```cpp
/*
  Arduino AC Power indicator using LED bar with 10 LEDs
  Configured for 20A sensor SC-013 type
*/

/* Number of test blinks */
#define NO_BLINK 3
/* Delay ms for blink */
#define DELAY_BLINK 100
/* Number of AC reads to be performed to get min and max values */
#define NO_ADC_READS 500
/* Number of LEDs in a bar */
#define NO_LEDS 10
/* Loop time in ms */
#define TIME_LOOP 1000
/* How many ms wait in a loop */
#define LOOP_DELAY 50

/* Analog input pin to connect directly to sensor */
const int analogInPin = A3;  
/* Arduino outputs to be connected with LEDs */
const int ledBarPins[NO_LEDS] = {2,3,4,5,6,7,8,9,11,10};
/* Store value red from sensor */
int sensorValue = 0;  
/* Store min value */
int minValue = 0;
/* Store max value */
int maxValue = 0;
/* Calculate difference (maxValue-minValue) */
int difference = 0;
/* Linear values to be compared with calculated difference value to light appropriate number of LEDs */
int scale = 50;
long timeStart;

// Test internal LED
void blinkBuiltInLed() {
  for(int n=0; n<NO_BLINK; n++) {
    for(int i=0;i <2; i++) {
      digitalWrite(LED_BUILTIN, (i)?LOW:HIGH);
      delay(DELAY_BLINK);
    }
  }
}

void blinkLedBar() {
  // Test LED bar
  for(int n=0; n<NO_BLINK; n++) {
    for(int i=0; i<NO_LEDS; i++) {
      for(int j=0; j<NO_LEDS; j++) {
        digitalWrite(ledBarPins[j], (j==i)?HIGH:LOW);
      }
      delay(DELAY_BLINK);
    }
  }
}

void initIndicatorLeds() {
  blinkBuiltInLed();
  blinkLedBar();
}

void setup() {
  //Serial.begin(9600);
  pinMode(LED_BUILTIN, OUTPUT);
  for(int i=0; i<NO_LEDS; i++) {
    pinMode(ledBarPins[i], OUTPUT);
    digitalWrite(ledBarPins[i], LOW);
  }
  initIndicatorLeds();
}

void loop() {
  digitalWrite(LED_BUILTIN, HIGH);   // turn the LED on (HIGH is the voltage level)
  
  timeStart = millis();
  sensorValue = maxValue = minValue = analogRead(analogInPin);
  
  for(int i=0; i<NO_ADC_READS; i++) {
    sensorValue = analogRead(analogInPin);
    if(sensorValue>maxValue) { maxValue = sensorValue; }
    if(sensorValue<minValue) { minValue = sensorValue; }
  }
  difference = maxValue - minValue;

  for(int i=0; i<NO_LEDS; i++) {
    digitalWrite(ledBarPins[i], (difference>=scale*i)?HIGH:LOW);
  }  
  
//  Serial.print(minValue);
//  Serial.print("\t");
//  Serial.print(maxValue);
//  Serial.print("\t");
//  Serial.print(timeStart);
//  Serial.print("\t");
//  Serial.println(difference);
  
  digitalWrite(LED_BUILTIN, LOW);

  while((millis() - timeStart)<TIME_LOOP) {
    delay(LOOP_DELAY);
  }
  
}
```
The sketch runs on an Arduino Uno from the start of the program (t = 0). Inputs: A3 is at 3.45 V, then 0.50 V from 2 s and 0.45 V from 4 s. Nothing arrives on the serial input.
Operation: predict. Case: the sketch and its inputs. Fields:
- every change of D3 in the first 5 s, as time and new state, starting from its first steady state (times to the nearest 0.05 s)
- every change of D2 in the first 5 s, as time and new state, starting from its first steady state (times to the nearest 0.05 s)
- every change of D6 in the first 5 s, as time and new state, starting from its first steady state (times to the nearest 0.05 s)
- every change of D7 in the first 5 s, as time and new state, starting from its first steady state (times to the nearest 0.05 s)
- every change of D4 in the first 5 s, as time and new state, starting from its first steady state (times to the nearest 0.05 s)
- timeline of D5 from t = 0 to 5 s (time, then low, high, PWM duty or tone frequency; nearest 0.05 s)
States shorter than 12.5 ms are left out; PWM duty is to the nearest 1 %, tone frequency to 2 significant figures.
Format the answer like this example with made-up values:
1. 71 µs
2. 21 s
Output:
1. 0 s low; 0.7 s high; 0.8 s low; 1.7 s high; 1.8 s low; 2.7 s high; 2.8 s low
2. 0 s low; 0.6 s high; 0.7 s low; 1.6 s high; 1.7 s low; 2.6 s high; 2.7 s low; 3.65 s high
3. 0 s low; 1 s high; 1.1 s low; 2 s high; 2.1 s low; 3 s high; 3.1 s low
4. 0 s low; 1.1 s high; 1.2 s low; 2.1 s high; 2.2 s low; 3.1 s high; 3.2 s low
5. 0 s low; 0.8 s high; 0.9 s low; 1.8 s high; 1.9 s low; 2.8 s high; 2.9 s low
6. 0 s low; 0.9 s high; 1 s low; 1.9 s high; 2 s low; 2.9 s high; 3 s low
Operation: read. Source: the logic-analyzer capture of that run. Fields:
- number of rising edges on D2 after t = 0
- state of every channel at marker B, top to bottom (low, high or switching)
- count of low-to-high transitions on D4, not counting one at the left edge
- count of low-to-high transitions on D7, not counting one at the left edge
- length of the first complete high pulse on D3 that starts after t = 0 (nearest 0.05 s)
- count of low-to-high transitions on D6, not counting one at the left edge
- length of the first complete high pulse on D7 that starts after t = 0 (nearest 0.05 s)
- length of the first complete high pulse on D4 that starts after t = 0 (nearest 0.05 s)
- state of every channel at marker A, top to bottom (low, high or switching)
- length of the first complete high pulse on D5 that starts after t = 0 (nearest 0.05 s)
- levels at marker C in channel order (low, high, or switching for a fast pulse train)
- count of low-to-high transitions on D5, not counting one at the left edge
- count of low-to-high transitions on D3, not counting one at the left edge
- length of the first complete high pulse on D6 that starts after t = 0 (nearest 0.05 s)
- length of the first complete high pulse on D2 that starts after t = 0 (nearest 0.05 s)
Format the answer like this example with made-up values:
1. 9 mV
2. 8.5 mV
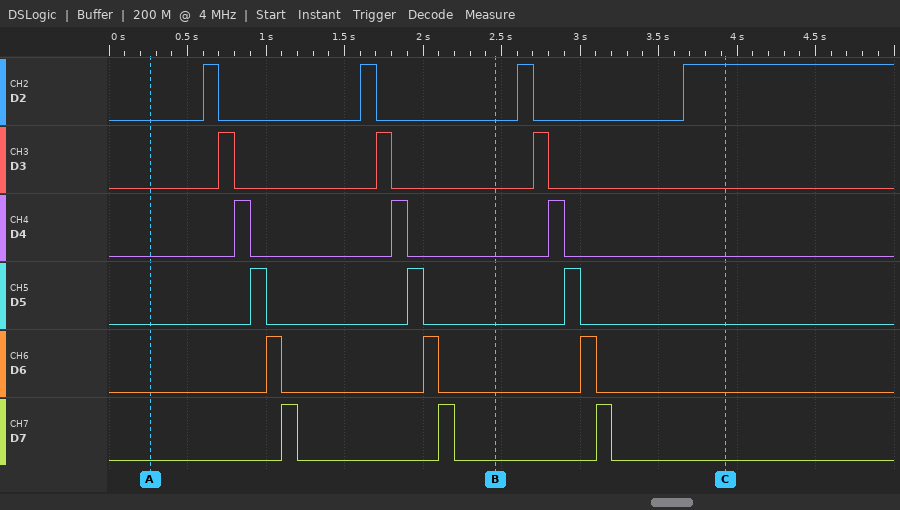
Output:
1. 4
2. D2 low, D3 low, D4 low, D5 low, D6 low, D7 low
3. 3
4. 3
5. 0.10 s
6. 3
7. 0.10 s
8. 0.10 s
9. D2 low, D3 low, D4 low, D5 low, D6 low, D7 low
10. 0.10 s
11. D2 high, D3 low, D4 low, D5 low, D6 low, D7 low
12. 3
13. 3
14. 0.10 s
15. 0.10 s
